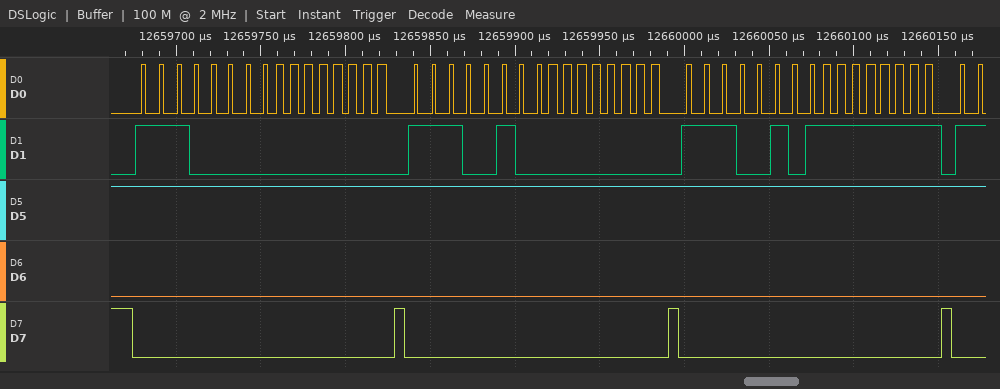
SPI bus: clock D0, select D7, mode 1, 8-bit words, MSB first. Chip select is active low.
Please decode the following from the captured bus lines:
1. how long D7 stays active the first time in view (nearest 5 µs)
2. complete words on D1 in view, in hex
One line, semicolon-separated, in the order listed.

155 µs; E0, 00, E4, 00, E5, FF
